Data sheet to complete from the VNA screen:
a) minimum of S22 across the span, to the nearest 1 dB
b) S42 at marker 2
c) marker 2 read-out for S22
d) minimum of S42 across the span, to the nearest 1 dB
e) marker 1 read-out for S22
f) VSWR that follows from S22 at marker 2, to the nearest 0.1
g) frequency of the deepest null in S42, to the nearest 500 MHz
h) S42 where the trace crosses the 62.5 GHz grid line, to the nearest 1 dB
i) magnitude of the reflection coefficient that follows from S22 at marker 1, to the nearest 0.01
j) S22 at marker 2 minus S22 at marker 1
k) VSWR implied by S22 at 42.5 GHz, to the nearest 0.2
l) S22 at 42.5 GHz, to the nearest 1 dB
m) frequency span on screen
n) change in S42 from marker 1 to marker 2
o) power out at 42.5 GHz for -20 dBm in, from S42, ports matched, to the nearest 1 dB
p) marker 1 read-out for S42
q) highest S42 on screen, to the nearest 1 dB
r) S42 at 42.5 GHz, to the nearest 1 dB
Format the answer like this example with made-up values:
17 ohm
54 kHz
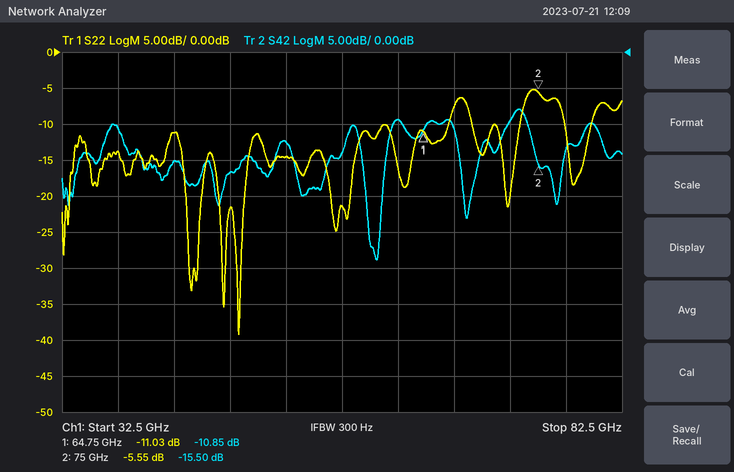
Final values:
-39 dB
-15.50 dB
-5.55 dB
-29 dB
-11.03 dB
3.2
60.5 GHz
-9 dB
0.28
5.48 dB
1.8
-11 dB
50 GHz
-4.65 dB
-35 dBm
-10.85 dB
-8 dB
-15 dB
